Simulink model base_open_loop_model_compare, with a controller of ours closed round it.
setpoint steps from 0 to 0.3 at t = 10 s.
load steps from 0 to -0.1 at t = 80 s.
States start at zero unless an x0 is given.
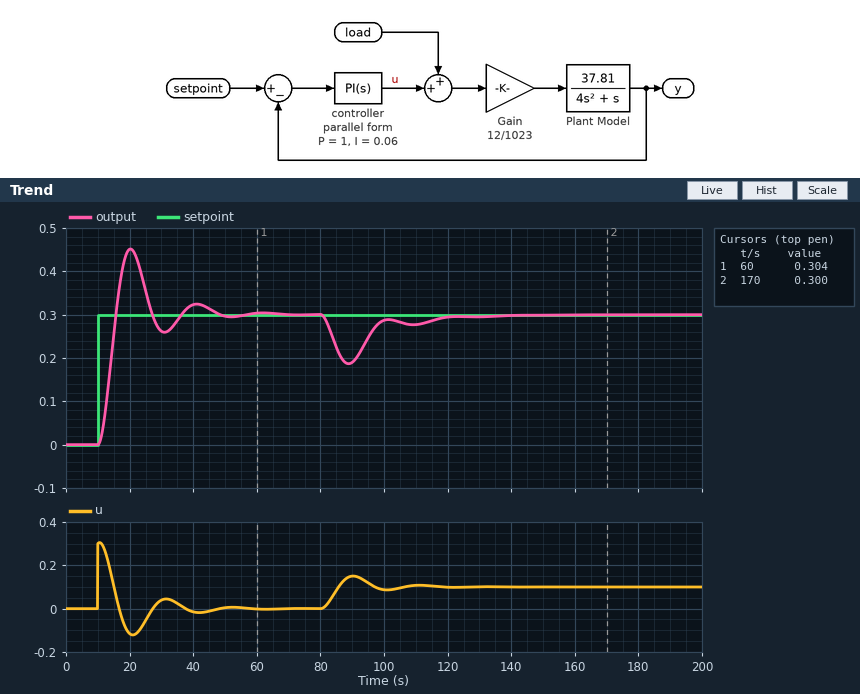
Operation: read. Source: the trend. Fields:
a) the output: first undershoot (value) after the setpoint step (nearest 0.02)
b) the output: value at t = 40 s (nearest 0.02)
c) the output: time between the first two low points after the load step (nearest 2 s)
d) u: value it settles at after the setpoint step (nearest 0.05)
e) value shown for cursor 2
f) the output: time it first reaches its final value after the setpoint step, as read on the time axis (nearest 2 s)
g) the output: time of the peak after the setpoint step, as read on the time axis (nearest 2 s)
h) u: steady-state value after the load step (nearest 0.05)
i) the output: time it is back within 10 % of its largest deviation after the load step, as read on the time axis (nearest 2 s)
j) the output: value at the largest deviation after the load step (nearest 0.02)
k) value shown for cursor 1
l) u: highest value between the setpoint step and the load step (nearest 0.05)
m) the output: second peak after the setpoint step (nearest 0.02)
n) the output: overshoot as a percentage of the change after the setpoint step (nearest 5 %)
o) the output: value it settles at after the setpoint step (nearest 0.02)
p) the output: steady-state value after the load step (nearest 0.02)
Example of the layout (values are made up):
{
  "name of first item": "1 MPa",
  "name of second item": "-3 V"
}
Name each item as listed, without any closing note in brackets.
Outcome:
{
  "the output: first undershoot (value) after the setpoint step": "0.26",
  "the output: value at t = 40 s": "0.32",
  "the output: time between the first two low points after the load step": "20 s",
  "u: value it settles at after the setpoint step": "0.00",
  "value shown for cursor 2": "0.300",
  "the output: time it first reaches its final value after the setpoint step, as read on the time axis": "16 s",
  "the output: time of the peak after the setpoint step, as read on the time axis": "20 s",
  "u: steady-state value after the load step": "0.10",
  "the output: time it is back within 10 % of its largest deviation after the load step, as read on the time axis": "116 s",
  "the output: value at the largest deviation after the load step": "0.18",
  "value shown for cursor 1": "0.304",
  "u: highest value between the setpoint step and the load step": "0.30",
  "the output: second peak after the setpoint step": "0.32",
  "the output: overshoot as a percentage of the change after the setpoint step": "50 %",
  "the output: value it settles at after the setpoint step": "0.30",
  "the output: steady-state value after the load step": "0.30"
}
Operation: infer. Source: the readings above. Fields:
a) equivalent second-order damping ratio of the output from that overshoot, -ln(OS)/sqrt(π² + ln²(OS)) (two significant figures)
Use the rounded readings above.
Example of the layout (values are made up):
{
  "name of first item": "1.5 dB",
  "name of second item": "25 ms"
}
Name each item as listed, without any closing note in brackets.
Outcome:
{
  "equivalent second-order damping ratio of the output from that overshoot, -ln(OS)/sqrt(π² + ln²(OS))": "0.22"
}
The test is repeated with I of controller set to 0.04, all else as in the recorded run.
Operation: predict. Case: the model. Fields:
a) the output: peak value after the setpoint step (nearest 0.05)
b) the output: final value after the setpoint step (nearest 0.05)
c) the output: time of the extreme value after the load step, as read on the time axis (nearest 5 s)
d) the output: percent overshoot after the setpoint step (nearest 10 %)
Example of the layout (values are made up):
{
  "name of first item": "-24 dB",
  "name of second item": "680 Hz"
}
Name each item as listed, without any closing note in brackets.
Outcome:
{
  "the output: peak value after the setpoint step": "0.45",
  "the output: final value after the setpoint step": "0.30",
  "the output: time of the extreme value after the load step, as read on the time axis": "90 s",
  "the output: percent overshoot after the setpoint step": "40 %"
}
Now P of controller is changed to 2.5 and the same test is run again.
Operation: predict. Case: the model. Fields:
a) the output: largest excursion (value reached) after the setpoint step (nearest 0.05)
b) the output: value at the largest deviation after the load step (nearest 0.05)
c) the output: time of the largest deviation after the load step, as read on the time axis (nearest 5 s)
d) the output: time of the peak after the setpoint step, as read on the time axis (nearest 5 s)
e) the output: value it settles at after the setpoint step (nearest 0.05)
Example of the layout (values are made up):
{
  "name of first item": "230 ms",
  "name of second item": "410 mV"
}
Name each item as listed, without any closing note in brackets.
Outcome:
{
  "the output: largest excursion (value reached) after the setpoint step": "0.45",
  "the output: value at the largest deviation after the load step": "0.25",
  "the output: time of the largest deviation after the load step, as read on the time axis": "85 s",
  "the output: time of the peak after the setpoint step, as read on the time axis": "15 s",
  "the output: value it settles at after the setpoint step": "0.30"
}
